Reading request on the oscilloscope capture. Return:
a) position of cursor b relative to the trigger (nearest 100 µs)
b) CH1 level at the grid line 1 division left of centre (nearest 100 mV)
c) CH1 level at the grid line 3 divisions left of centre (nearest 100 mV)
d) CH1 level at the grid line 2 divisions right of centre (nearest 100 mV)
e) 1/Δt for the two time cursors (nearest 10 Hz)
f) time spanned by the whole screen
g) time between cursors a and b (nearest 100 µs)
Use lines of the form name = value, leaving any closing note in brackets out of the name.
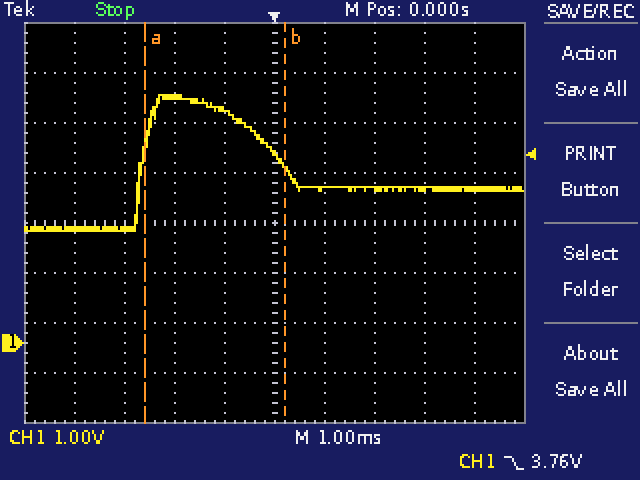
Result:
position of cursor b relative to the trigger = +200 µs
CH1 level at the grid line 1 division left of centre = 4.7 V
CH1 level at the grid line 3 divisions left of centre = 2.3 V
CH1 level at the grid line 2 divisions right of centre = 3.1 V
1/Δt for the two time cursors = 360 Hz
time spanned by the whole screen = 10 ms
time between cursors a and b = 2.8 ms
